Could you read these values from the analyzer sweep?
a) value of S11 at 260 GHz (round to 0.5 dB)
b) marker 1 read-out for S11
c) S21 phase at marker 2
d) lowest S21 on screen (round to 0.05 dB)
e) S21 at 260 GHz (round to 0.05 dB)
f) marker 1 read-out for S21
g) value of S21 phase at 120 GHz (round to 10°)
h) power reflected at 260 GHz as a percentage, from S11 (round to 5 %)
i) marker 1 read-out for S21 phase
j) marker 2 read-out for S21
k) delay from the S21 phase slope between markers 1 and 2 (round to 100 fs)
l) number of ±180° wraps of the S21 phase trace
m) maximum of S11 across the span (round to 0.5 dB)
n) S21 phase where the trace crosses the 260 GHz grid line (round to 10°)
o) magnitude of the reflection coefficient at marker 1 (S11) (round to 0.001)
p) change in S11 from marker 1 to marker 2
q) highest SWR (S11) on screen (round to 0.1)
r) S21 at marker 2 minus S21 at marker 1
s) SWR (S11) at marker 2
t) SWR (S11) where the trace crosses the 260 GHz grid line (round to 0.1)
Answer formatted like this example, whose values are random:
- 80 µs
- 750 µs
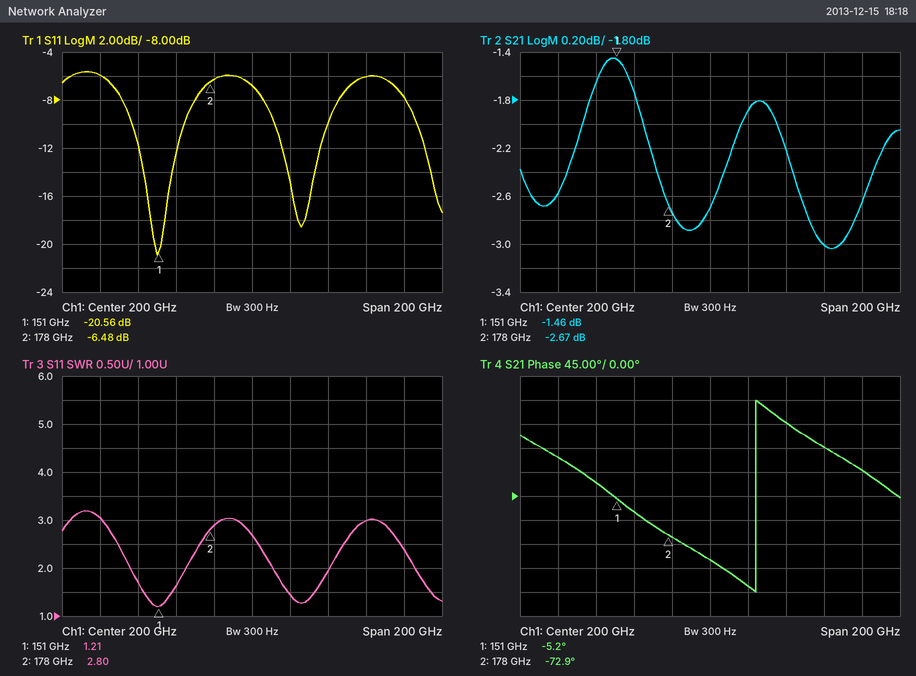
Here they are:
- -6.0 dB
- -20.56 dB
- -72.9°
- -3.05 dB
- -3.00 dB
- -1.46 dB
- 70°
- 25 %
- -5.2°
- -2.67 dB
- 7.0 ps
- 1
- -5.5 dB
- 90°
- 0.094
- 14.08 dB
- 3.2
- -1.21 dB
- 2.80
- 3.0
